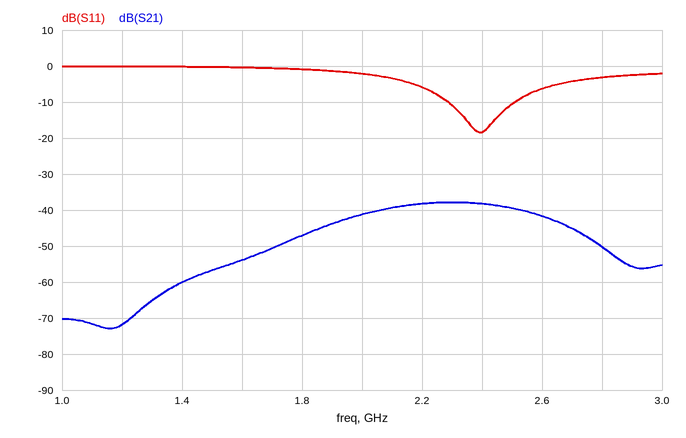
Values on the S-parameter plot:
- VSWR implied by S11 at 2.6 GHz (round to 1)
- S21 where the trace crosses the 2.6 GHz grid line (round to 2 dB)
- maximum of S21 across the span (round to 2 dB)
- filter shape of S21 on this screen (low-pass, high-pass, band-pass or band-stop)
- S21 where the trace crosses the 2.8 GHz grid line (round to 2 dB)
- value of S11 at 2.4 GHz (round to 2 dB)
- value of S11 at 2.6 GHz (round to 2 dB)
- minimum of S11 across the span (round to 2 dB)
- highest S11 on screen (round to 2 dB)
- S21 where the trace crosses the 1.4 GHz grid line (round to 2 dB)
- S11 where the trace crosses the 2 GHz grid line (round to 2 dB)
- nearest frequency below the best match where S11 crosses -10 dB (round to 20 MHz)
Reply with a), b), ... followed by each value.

a) 3
b) -42 dB
c) -38 dB
d) band-pass
e) -50 dB
f) -18 dB
g) -6 dB
h) -18 dB
i) 0 dB
j) -60 dB
k) -2 dB
l) 2.28 GHz
